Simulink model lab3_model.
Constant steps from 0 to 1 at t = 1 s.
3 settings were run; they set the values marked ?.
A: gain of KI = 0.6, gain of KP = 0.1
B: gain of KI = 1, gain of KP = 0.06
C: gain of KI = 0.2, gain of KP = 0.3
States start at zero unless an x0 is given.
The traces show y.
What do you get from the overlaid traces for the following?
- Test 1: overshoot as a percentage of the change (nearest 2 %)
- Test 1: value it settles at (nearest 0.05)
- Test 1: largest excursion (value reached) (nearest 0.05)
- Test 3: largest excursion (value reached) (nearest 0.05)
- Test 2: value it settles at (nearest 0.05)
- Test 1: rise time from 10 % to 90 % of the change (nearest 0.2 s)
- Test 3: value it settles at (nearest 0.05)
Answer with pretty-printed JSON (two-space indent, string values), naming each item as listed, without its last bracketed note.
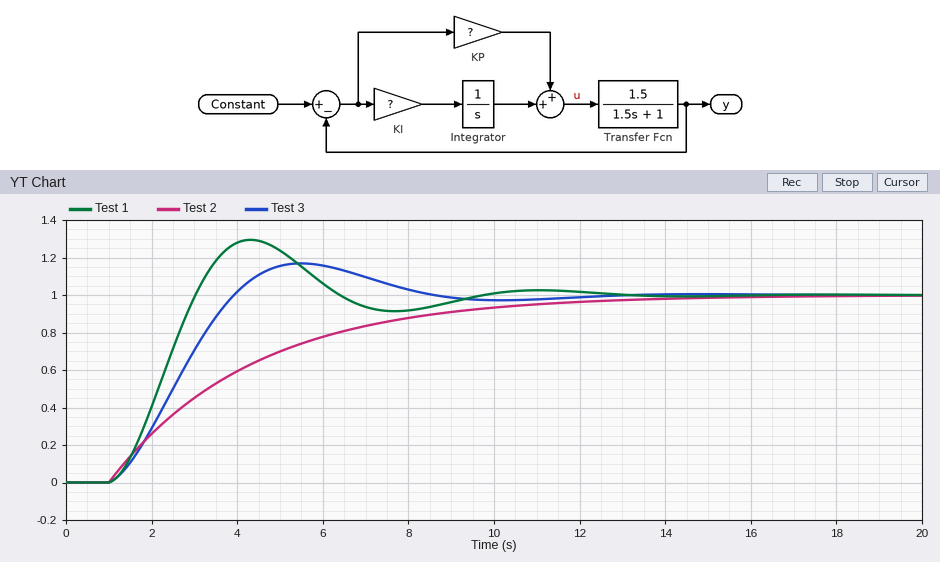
{
  "Test 1: overshoot as a percentage of the change": "30 %",
  "Test 1: value it settles at": "1.00",
  "Test 1: largest excursion (value reached)": "1.30",
  "Test 3: largest excursion (value reached)": "1.15",
  "Test 2: value it settles at": "1.00",
  "Test 1: rise time from 10 % to 90 % of the change": "1.4 s",
  "Test 3: value it settles at": "1.00"
}
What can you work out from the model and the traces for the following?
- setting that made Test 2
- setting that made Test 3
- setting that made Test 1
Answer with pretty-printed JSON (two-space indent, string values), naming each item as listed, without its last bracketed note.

{
  "setting that made Test 2": "C",
  "setting that made Test 3": "A",
  "setting that made Test 1": "B"
}
